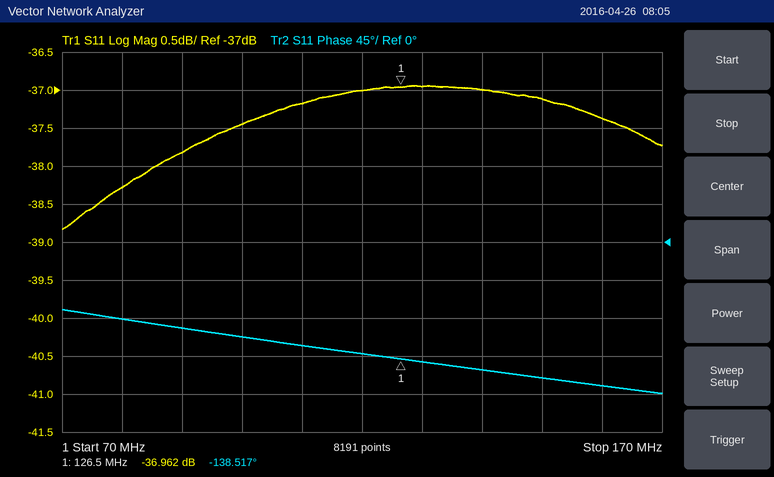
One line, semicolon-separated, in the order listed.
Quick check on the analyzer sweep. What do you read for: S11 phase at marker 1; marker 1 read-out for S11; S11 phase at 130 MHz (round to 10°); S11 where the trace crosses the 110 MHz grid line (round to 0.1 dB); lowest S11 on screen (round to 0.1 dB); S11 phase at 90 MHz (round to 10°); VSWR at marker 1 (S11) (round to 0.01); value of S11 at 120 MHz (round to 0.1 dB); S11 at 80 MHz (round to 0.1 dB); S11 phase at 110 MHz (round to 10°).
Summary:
-138.517°; -36.962 dB; -140°; -37.2 dB; -38.8 dB; -100°; 1.03; -37.0 dB; -38.3 dB; -120°
